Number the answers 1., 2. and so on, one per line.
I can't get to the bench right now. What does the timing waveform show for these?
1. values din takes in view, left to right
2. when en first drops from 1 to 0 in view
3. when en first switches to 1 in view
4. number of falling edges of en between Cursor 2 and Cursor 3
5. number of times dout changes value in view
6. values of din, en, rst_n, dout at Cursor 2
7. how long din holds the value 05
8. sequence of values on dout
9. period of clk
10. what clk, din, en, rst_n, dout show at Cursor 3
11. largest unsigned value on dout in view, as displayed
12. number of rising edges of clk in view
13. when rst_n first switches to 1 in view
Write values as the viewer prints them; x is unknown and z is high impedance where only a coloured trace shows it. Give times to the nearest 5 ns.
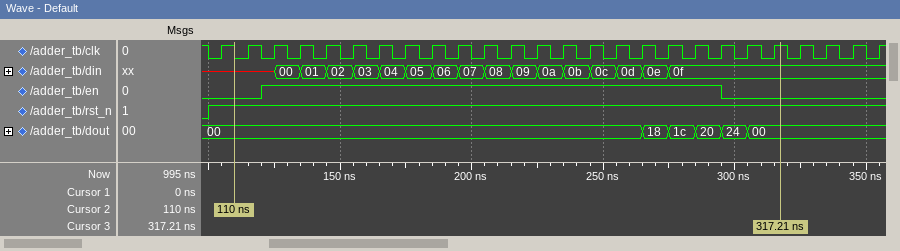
1. x, 00, 01, 02, 03, 04, 05, 06, 07, 08, 09, 0a, 0b, 0c, 0d, 0e, 0f
2. 295 ns
3. 120 ns
4. 1
5. 5
6. din=x, en=0, rst_n=1, dout=00
7. 10 ns
8. 00, 18, 1c, 20, 24, 00
9. 10 ns
10. clk=1, din=0f, en=0, rst_n=1, dout=00
11. 24
12. 26
13. 100 ns
